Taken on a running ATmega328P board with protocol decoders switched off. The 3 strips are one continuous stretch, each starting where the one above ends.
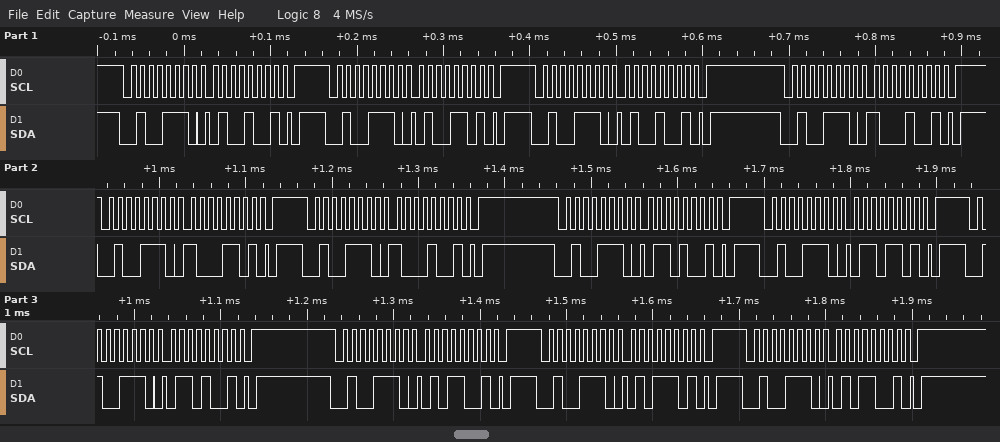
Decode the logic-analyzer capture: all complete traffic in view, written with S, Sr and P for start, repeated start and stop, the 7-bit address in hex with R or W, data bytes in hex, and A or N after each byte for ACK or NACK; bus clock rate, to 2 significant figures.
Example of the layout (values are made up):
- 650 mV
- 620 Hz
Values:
- S 27W A 49 A P S 27W A 4D A P S 27W A 49 A P S 27W A 89 A P S 27W A 8D A P S 27W A 89 A P S 27W A 69 A P S 27W A 6D A P S 27W A 69 A P S 27W A 59 A P S 27W A 5D A P S 27W A 59 A P
- 100 kHz
